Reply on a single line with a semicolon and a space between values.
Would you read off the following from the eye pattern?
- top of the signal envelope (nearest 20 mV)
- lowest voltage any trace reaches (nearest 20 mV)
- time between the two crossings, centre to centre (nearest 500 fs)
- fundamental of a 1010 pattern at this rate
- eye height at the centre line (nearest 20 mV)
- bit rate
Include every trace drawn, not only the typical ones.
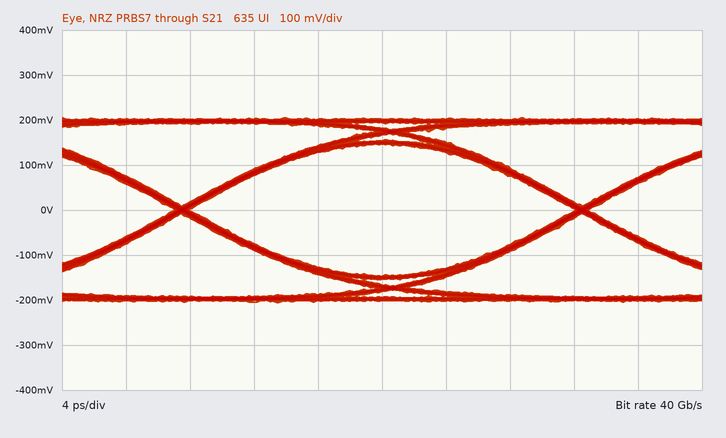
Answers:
200 mV; -200 mV; 25.0 ps; 20 GHz; 300 mV; 40 Gb/s
